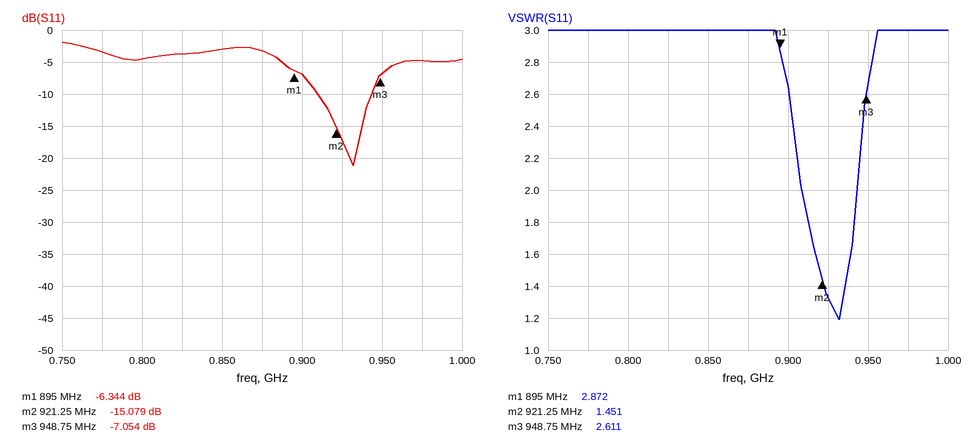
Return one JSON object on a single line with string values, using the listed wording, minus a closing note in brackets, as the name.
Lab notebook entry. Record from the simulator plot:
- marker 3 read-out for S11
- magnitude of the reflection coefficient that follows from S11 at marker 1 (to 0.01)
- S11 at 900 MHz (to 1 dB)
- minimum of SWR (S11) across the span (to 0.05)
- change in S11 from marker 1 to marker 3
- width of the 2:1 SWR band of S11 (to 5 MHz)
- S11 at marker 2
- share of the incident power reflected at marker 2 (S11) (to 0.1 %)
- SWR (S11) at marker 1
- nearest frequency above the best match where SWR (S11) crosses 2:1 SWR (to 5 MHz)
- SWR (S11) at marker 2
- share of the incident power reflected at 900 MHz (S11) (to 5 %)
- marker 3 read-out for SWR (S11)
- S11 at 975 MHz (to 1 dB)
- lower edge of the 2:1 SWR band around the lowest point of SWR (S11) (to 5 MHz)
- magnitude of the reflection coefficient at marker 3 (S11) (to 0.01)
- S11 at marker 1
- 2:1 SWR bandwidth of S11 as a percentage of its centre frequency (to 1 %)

{"marker 3 read-out for S11": "-7.054 dB", "magnitude of the reflection coefficient that follows from S11 at marker 1": "0.48", "S11 at 900 MHz": "-7 dB", "minimum of SWR (S11) across the span": "1.20", "change in S11 from marker 1 to marker 3": "-0.710 dB", "width of the 2:1 SWR band of S11": "35 MHz", "S11 at marker 2": "-15.079 dB", "share of the incident power reflected at marker 2 (S11)": "3.1 %", "SWR (S11) at marker 1": "2.872", "nearest frequency above the best match where SWR (S11) crosses 2:1 SWR": "945 MHz", "SWR (S11) at marker 2": "1.451", "share of the incident power reflected at 900 MHz (S11)": "20 %", "marker 3 read-out for SWR": "2.611", "S11 at 975 MHz": "-5 dB", "lower edge of the 2:1 SWR band around the lowest point of SWR (S11)": "910 MHz", "magnitude of the reflection coefficient at marker 3 (S11)": "0.44", "S11 at marker 1": "-6.344 dB", "2:1 SWR bandwidth of S11 as a percentage of its centre frequency": "4 %"}
